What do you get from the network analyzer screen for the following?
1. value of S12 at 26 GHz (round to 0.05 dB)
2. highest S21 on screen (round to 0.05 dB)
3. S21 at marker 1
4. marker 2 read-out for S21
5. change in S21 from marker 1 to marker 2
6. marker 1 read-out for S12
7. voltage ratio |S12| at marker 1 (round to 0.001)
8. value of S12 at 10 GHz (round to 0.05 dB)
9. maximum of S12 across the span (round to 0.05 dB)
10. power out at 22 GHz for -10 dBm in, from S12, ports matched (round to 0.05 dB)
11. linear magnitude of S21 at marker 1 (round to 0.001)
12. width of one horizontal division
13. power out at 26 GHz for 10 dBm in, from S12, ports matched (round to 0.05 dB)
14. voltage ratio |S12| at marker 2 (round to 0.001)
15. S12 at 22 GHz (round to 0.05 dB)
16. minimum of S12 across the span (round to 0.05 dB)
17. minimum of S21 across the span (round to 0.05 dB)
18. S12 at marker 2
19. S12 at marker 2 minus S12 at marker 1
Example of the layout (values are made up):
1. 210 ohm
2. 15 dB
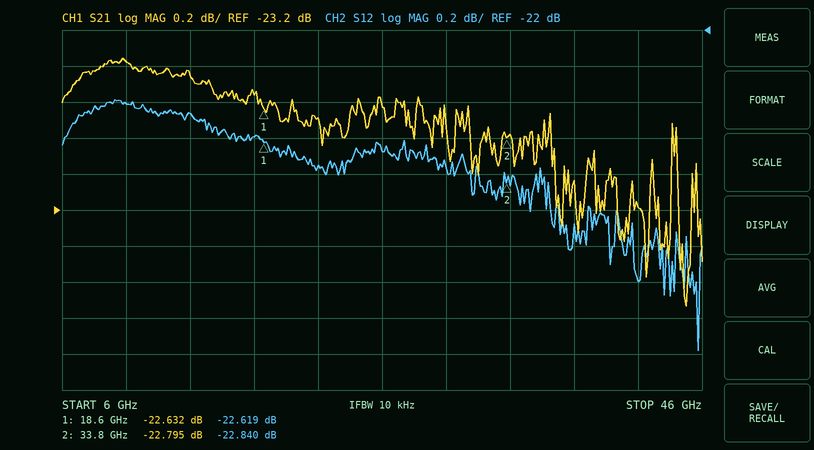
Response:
1. -22.65 dB
2. -22.35 dB
3. -22.632 dB
4. -22.795 dB
5. -0.163 dB
6. -22.619 dB
7. 0.074
8. -22.40 dB
9. -22.40 dB
10. -32.75 dBm
11. 0.074
12. 4 GHz
13. -12.65 dBm
14. 0.072
15. -22.75 dB
16. -23.80 dB
17. -23.75 dB
18. -22.840 dB
19. -0.221 dB
